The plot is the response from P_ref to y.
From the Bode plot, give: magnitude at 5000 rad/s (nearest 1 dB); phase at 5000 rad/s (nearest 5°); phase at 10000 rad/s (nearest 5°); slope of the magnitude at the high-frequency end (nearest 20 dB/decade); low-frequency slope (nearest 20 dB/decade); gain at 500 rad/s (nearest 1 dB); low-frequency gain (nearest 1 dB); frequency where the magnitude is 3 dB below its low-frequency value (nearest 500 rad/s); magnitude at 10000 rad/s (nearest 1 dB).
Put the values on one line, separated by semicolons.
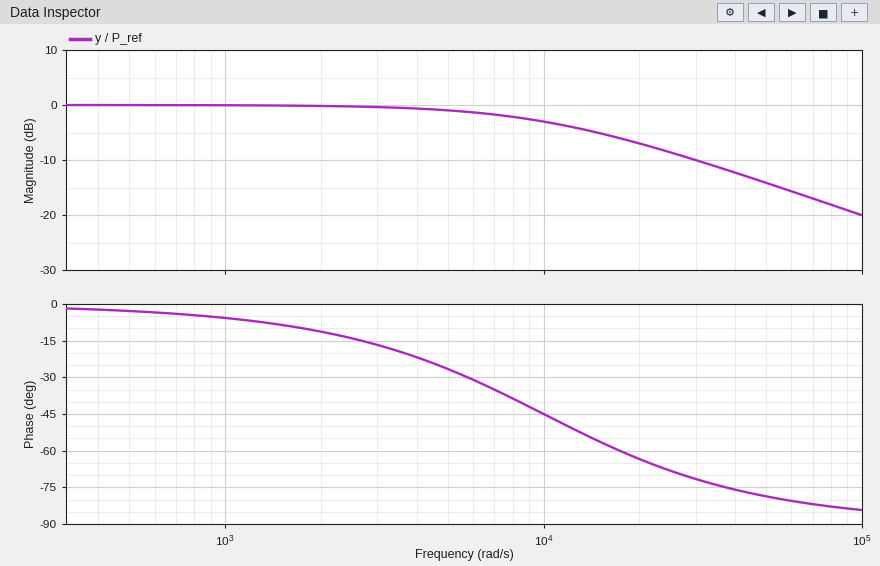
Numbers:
-1 dB; -25°; -45°; -20 dB/decade; 0 dB/decade; 0 dB; 0 dB; 10000 rad/s; -3 dB
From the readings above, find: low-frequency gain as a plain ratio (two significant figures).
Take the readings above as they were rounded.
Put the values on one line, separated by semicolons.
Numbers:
1.0
